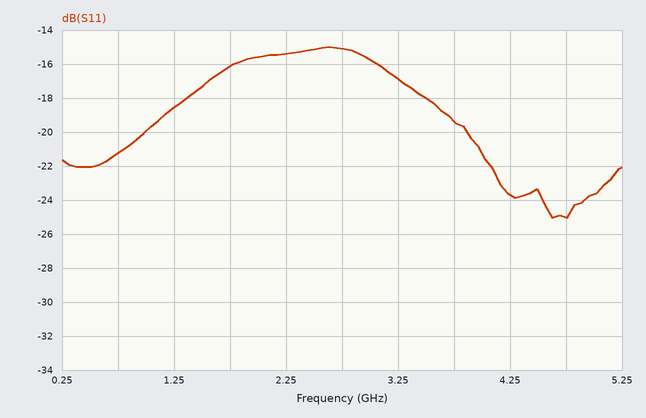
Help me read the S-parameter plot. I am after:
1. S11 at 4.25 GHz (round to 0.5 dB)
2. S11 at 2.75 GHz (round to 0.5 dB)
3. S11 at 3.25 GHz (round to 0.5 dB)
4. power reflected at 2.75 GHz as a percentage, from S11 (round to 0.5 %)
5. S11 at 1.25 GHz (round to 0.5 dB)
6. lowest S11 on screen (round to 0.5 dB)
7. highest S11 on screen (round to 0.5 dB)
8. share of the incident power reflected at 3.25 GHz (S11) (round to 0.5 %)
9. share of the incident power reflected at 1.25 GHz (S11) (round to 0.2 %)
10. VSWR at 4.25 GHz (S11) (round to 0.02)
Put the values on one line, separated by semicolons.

-23.5 dB; -15.0 dB; -17.0 dB; 3.0 %; -18.5 dB; -25.0 dB; -15.0 dB; 2.0 %; 1.4 %; 1.14
